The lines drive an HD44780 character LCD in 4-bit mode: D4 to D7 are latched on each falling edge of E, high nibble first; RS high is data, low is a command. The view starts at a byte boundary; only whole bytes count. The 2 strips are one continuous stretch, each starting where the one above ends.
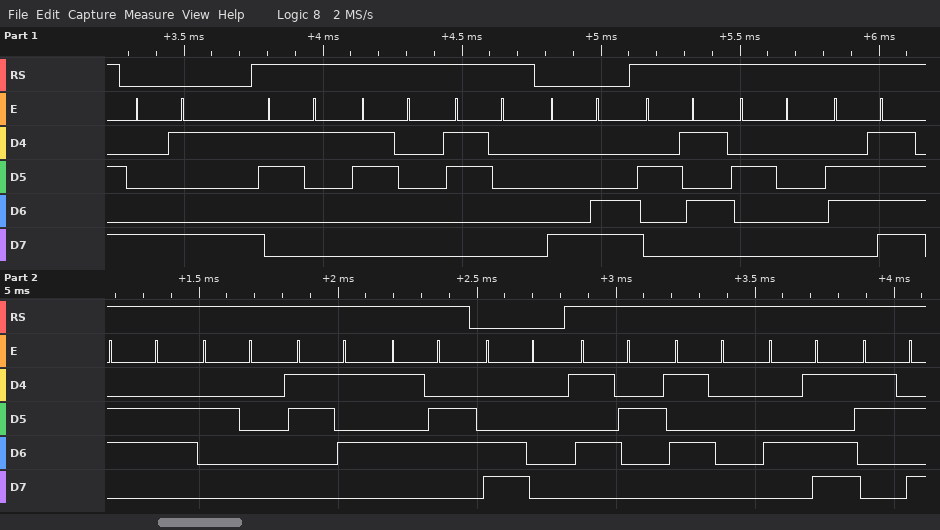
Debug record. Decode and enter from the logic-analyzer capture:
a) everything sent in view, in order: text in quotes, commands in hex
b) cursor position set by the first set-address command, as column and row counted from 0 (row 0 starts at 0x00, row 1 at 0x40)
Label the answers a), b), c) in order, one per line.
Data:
a) 0x89 "100" 0x8C "% of 5V" 0xC0 "RPM:"
b) column 9, row 0
